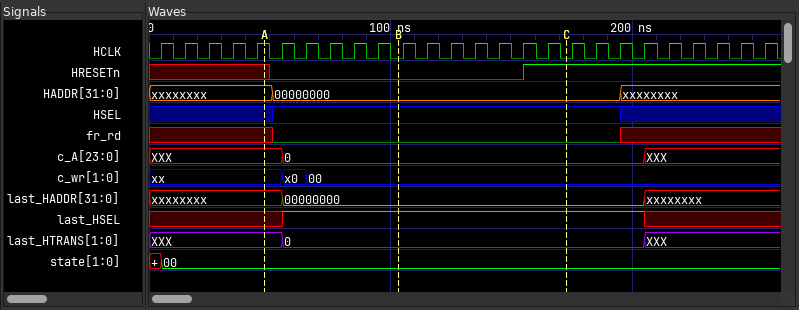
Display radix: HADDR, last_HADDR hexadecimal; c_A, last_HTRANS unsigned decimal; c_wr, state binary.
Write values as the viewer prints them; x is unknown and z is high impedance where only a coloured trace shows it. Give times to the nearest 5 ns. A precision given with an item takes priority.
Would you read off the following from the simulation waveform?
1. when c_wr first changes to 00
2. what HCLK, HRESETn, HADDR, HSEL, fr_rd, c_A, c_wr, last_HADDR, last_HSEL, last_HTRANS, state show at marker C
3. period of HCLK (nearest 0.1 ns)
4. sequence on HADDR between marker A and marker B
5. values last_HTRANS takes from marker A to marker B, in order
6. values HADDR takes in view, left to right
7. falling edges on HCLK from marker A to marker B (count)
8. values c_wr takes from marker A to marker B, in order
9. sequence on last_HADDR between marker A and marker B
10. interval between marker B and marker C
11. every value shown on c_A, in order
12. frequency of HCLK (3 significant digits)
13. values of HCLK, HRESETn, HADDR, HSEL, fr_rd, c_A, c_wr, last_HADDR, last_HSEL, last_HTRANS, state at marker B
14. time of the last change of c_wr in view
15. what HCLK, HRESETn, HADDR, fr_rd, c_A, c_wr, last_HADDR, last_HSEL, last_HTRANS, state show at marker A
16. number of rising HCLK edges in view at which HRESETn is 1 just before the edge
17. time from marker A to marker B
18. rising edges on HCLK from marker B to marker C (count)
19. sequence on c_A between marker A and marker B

65 ns
HCLK=0, HRESETn=1, HADDR=00000000, HSEL=1, fr_rd=0, c_A=0, c_wr=00, last_HADDR=00000000, last_HSEL=1, last_HTRANS=0, state=00
10 ns
xxxxxxxx, 00000000
XXX, 0
xxxxxxxx, 00000000, xxxxxxxx
6
xx, x0, 00
xxxxxxxx, 00000000
70 ns
XXX, 0, XXX
100 MHz
HCLK=0, HRESETn=0, HADDR=00000000, HSEL=1, fr_rd=0, c_A=0, c_wr=00, last_HADDR=00000000, last_HSEL=1, last_HTRANS=0, state=00
65 ns
HCLK=1, HRESETn=x, HADDR=xxxxxxxx, fr_rd=x, c_A=XXX, c_wr=xx, last_HADDR=xxxxxxxx, last_HSEL=x, last_HTRANS=XXX, state=00
10
55 ns
7
XXX, 0
